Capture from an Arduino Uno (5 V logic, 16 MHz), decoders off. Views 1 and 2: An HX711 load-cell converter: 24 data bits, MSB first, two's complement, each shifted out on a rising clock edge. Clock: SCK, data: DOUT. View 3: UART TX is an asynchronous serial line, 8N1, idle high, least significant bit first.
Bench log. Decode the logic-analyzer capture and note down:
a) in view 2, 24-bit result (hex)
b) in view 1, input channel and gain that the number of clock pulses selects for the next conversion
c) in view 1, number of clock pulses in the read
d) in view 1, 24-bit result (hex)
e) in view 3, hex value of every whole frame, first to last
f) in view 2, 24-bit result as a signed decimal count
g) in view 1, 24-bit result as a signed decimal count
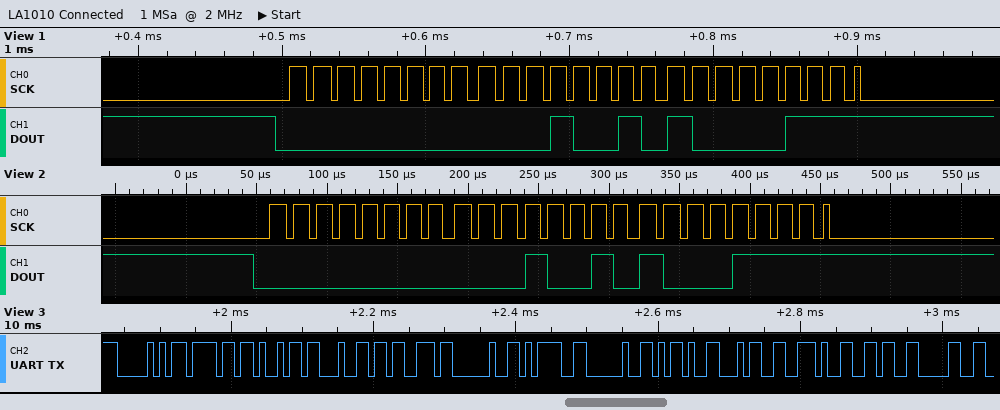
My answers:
0x00128F
channel A, gain 128
25
0x001287
50 6F 69 64 73 20 3D 20 2D 34 2E 36 30
4751
4743
